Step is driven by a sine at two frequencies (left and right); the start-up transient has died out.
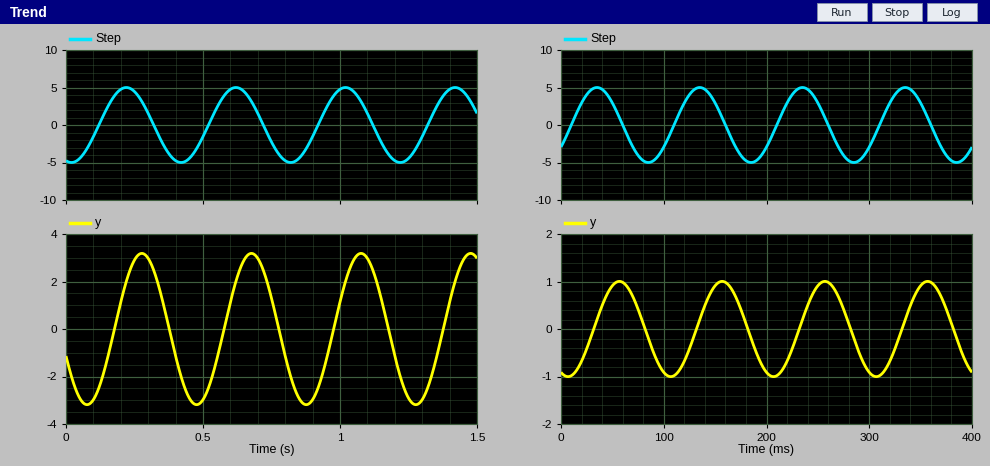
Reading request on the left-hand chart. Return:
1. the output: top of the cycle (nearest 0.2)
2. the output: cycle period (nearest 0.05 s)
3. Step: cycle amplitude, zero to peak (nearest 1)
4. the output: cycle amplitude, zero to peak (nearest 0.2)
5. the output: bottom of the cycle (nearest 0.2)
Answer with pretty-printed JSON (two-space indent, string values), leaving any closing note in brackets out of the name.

{
  "the output: top of the cycle": "3.2",
  "the output: cycle period": "0.40 s",
  "Step: cycle amplitude, zero to peak": "5",
  "the output: cycle amplitude, zero to peak": "3.2",
  "the output: bottom of the cycle": "-3.2"
}
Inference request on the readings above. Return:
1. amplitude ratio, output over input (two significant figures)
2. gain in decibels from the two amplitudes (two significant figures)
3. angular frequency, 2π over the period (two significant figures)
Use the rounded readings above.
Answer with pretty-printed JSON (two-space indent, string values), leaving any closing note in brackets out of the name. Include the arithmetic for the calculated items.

{
  "amplitude ratio, output over input": "3.2 / 5 = 0.64",
  "gain in decibels from the two amplitudes": "20 log10(3.2 / 5) = -3.9 dB",
  "angular frequency, 2π over the period": "2π / 0.4 = 16 rad/s"
}
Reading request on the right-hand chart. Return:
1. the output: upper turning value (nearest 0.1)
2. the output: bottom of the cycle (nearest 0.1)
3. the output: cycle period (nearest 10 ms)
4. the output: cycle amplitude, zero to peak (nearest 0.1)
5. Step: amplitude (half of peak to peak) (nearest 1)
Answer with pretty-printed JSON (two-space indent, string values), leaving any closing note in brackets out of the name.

{
  "the output: upper turning value": "1.0",
  "the output: bottom of the cycle": "-1.0",
  "the output: cycle period": "100 ms",
  "the output: cycle amplitude, zero to peak": "1.0",
  "Step: amplitude (half of peak to peak)": "5"
}
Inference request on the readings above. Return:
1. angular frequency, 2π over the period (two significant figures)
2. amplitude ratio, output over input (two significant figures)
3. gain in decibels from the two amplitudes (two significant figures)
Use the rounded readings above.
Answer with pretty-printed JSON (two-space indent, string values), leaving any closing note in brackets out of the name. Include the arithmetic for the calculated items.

{
  "angular frequency, 2π over the period": "2π / 100 = 0.063 rad/ms",
  "amplitude ratio, output over input": "1 / 5 = 0.20",
  "gain in decibels from the two amplitudes": "20 log10(1 / 5) = -14 dB"
}
